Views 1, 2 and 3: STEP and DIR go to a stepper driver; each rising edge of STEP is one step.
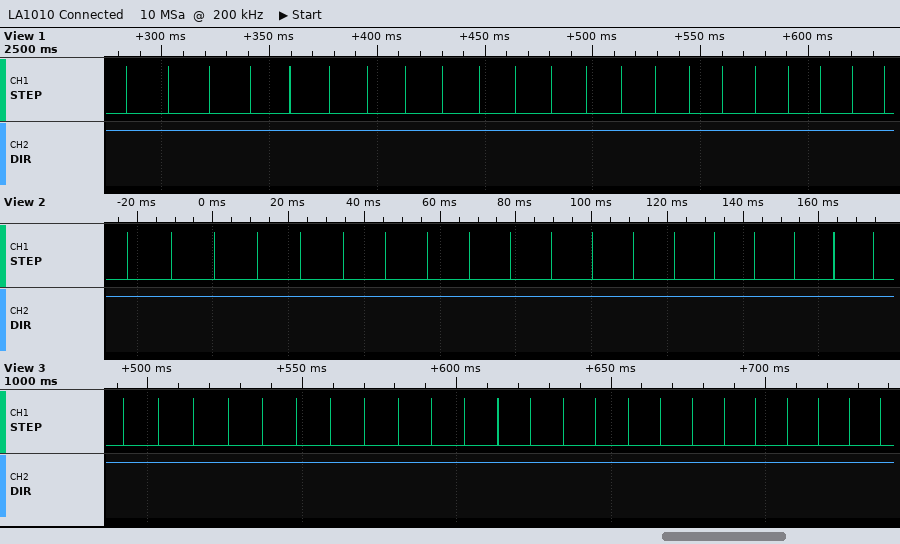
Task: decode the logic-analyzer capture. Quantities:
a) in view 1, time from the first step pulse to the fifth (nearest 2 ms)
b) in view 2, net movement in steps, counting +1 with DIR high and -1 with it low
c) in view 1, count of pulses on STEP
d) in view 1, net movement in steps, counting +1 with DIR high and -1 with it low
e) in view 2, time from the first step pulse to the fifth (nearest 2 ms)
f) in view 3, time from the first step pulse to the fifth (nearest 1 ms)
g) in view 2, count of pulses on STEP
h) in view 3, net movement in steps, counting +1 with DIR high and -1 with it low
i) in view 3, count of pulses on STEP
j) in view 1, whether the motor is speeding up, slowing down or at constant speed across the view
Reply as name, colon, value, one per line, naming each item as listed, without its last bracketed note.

in view 1, time from the first step pulse to the fifth: 76 ms
in view 2, net movement in steps, counting +1 with DIR high and -1 with it low: +19
in view 1, count of pulses on STEP: 22
in view 1, net movement in steps, counting +1 with DIR high and -1 with it low: +22
in view 2, time from the first step pulse to the fifth: 46 ms
in view 3, time from the first step pulse to the fifth: 45 ms
in view 2, count of pulses on STEP: 19
in view 3, net movement in steps, counting +1 with DIR high and -1 with it low: +24
in view 3, count of pulses on STEP: 24
in view 1, whether the motor is speeding up, slowing down or at constant speed across the view: speeding up
